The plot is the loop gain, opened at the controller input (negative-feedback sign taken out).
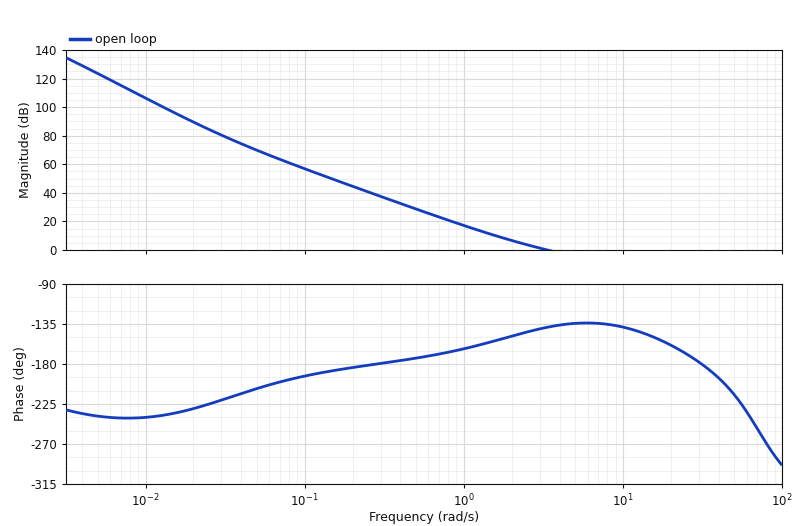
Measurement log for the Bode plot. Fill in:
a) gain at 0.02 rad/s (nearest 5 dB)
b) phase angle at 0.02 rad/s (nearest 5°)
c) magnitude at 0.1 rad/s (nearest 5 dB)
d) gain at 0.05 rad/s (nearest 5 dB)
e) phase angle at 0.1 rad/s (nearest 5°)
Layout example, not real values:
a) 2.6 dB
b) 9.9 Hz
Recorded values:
a) 90 dB
b) -230°
c) 55 dB
d) 70 dB
e) -195°
